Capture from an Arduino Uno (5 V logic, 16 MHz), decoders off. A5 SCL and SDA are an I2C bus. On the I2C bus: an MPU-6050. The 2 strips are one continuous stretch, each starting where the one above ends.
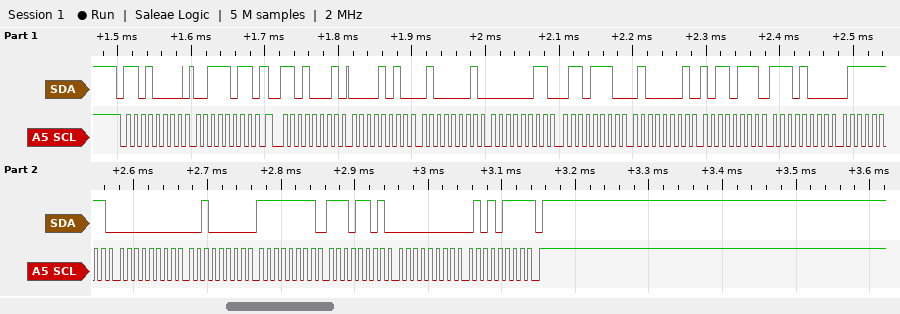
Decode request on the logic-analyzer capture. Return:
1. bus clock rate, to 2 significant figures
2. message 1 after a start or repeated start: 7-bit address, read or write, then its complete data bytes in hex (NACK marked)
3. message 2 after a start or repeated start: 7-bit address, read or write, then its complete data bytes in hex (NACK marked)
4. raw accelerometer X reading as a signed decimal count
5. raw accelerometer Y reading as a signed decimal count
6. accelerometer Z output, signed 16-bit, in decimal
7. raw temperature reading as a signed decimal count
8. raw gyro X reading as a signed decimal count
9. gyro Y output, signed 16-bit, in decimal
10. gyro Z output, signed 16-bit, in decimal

100 kHz
0x68 write: 3B
0x68 read: 0A 41 03 6E 41 B7 E8 7F 00 20 FF ED 00 57 NACK
2625
878
16823
-6017
32
-19
87
